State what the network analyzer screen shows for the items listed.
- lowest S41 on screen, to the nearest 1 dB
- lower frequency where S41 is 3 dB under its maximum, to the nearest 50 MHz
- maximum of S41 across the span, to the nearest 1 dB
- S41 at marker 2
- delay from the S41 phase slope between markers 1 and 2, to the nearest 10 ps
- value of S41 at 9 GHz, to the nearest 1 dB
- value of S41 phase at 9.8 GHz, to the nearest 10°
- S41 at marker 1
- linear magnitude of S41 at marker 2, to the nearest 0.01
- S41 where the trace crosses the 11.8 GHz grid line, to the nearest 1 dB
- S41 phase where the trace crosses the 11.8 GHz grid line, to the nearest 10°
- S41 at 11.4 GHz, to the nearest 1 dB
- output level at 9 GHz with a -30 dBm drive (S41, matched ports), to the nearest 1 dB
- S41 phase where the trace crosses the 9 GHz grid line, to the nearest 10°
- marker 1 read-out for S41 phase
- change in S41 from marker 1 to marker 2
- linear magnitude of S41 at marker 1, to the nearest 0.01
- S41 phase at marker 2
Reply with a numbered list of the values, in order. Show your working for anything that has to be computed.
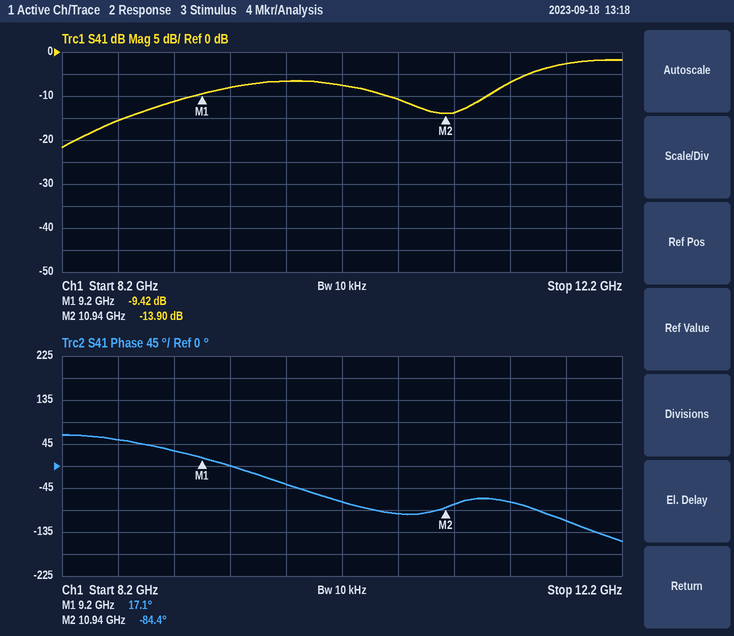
1. -22 dB
2. 11.55 GHz
3. -2 dB
4. -13.90 dB
5. −(-84.4° − (17.1°))/(360° × 1.74 GHz) ≈ 162 ps, so 160 ps to the nearest 10 ps
6. -11 dB
7. -40°
8. -9.42 dB
9. 10^(-13.9/20) ≈ 0.20
10. -3 dB
11. -110°
12. -7 dB
13. -30 dBm + (-11 dB) = -41 dBm
14. 30°
15. 17.1°
16. -13.9 − (-9.42) = -4.48 dB
17. 10^(-9.42/20) ≈ 0.34
18. -84.4°
